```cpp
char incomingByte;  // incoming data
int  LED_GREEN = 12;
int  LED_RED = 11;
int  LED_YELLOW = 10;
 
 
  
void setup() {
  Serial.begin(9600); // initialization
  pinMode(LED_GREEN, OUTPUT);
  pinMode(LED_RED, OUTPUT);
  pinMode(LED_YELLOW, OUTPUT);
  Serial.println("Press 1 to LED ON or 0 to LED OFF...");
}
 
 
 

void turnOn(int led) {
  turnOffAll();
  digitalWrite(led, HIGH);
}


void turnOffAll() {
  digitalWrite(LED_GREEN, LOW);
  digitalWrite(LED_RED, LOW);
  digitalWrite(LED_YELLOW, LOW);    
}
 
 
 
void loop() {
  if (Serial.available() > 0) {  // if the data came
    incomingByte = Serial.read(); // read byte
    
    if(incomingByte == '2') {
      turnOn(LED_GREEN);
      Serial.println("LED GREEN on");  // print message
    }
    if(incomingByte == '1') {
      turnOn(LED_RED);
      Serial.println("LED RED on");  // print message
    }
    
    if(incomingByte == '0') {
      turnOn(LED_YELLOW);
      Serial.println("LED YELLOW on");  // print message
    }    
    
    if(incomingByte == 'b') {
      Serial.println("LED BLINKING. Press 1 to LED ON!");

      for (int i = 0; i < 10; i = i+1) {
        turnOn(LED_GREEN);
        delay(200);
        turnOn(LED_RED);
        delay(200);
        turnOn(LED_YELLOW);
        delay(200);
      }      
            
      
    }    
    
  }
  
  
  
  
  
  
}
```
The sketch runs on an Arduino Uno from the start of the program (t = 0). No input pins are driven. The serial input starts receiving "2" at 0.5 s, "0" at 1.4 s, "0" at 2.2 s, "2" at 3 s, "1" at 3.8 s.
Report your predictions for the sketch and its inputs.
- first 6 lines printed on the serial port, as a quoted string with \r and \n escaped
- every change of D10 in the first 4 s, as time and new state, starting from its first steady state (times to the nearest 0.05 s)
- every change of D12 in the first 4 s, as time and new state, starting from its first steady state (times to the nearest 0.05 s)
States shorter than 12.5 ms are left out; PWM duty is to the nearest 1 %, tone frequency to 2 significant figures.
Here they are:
"Press 1 to LED ON or 0 to LED OFF...\r\nLED GREEN on\r\nLED YELLOW on\r\nLED YELLOW on\r\nLED GREEN on\r\nLED RED on\r\n"
0 s low; 1.4 s high; 3 s low
0 s low; 0.5 s high; 1.4 s low; 3 s high; 3.8 s low
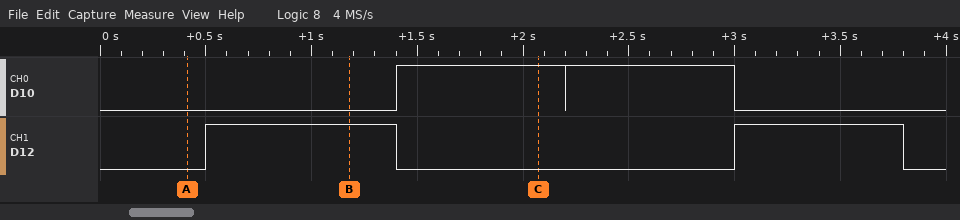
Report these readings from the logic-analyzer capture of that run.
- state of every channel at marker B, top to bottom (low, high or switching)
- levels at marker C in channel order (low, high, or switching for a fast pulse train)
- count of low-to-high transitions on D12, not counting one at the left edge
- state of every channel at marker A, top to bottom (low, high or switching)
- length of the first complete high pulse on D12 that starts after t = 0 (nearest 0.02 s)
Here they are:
D10 low, D12 high
D10 high, D12 low
2
D10 low, D12 low
0.90 s
